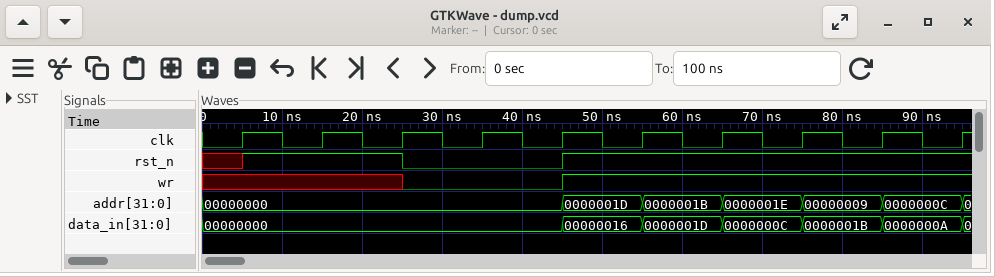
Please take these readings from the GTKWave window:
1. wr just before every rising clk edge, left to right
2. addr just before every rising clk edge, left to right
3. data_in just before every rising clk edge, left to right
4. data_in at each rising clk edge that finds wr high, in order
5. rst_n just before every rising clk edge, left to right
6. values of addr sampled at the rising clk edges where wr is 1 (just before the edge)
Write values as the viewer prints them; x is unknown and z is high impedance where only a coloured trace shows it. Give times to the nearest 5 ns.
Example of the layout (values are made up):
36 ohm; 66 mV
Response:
x x x 0 0 1 1 1 1 1; 00000000, 00000000, 00000000, 00000000, 00000000, 0000001D, 0000001B, 0000001E, 00000009, 0000000C; 00000000, 00000000, 00000000, 00000000, 00000000, 00000016, 0000001D, 0000000C, 0000001B, 0000000A; 00000016, 0000001D, 0000000C, 0000001B, 0000000A; x 1 1 0 0 1 1 1 1 1; 0000001D, 0000001B, 0000001E, 00000009, 0000000C
